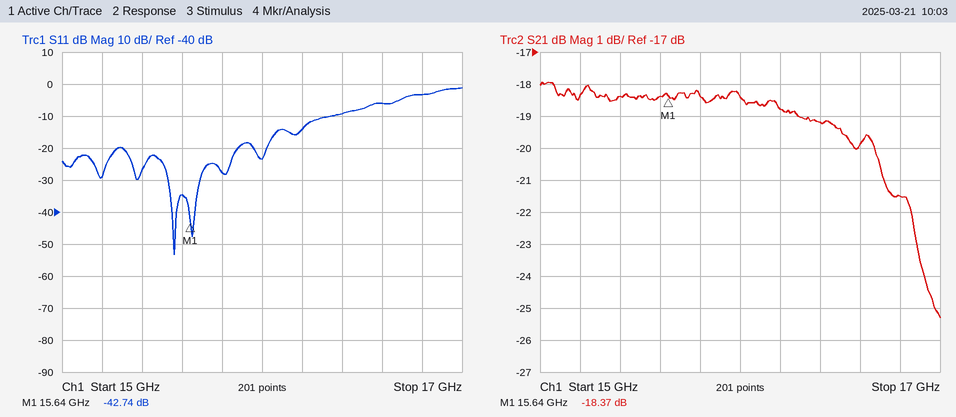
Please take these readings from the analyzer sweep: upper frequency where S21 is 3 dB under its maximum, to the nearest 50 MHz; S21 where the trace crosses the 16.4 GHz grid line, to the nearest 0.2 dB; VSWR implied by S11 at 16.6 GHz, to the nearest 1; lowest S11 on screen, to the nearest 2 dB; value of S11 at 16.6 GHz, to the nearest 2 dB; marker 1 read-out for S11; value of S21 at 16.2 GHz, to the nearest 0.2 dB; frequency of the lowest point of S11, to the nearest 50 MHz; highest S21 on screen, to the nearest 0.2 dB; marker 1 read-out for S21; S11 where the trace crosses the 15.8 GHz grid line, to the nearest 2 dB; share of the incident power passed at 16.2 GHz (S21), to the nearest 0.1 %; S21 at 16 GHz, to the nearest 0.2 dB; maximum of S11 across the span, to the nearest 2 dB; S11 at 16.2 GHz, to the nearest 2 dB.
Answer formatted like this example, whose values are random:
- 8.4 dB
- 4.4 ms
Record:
- 16.70 GHz
- -19.2 dB
- 3
- -54 dB
- -6 dB
- -42.74 dB
- -18.8 dB
- 15.55 GHz
- -18.0 dB
- -18.37 dB
- -28 dB
- 1.3 %
- -18.4 dB
- -2 dB
- -14 dB
